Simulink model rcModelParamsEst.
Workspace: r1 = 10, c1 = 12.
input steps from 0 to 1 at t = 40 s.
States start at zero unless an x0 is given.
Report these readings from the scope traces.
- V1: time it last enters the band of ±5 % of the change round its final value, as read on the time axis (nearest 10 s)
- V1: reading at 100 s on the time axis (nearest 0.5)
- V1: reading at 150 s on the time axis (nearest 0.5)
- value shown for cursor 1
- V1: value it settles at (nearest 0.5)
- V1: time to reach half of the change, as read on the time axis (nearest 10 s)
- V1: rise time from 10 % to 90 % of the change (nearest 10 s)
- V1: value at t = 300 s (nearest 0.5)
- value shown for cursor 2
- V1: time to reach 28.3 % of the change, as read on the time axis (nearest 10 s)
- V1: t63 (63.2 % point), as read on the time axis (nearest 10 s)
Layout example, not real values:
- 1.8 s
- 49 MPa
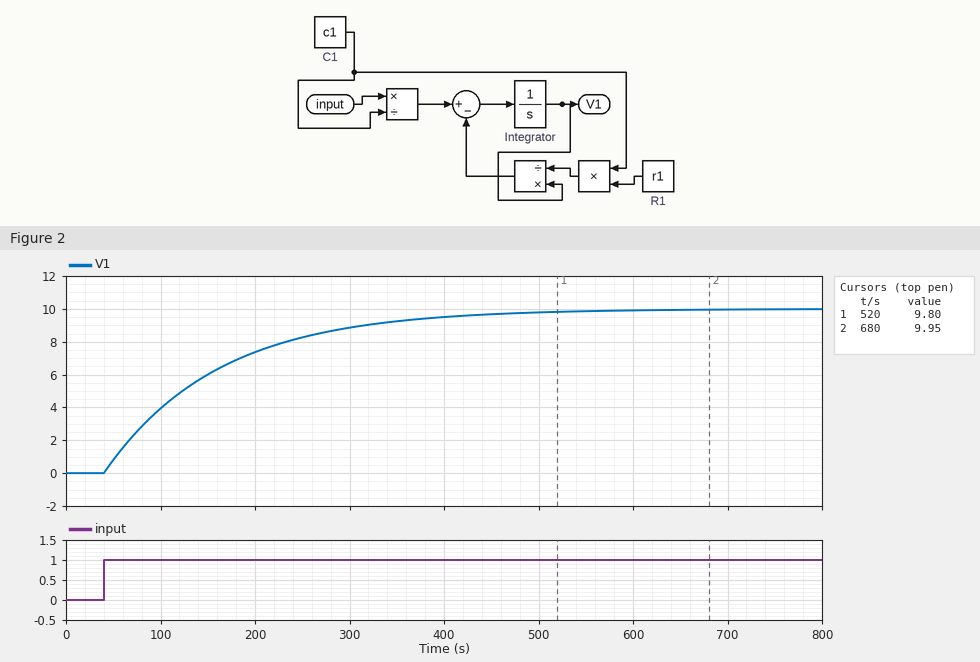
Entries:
- 400 s
- 4.0
- 6.0
- 9.80
- 10.0
- 120 s
- 260 s
- 9.0
- 9.95
- 80 s
- 160 s
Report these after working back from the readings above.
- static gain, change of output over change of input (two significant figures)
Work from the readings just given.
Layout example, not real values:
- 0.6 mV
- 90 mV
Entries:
- 10
